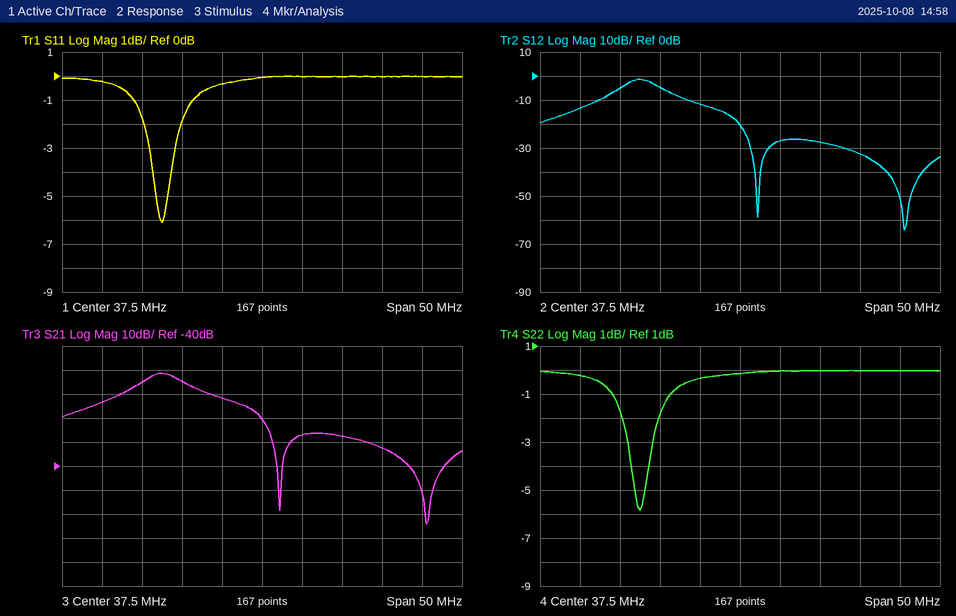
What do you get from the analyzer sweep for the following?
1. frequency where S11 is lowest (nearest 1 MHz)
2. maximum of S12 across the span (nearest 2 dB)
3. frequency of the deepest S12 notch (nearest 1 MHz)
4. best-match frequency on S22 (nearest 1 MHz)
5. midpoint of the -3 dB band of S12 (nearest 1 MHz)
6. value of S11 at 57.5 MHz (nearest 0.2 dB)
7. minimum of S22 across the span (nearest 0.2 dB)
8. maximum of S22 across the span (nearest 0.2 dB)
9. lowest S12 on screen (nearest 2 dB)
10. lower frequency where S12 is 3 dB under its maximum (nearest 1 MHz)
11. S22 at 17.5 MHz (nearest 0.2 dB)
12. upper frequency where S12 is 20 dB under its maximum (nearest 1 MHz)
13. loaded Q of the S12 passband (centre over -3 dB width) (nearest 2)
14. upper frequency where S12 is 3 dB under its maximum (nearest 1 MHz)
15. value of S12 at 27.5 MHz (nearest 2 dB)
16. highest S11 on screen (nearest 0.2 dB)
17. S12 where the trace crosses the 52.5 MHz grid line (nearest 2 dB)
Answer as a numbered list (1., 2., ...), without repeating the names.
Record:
1. 25 MHz
2. -2 dB
3. 58 MHz
4. 25 MHz
5. 25 MHz
6. 0.0 dB
7. -5.8 dB
8. 0.0 dB
9. -64 dB
10. 23 MHz
11. -0.2 dB
12. 38 MHz
13. 6
14. 27 MHz
15. -4 dB
16. 0.0 dB
17. -32 dB
